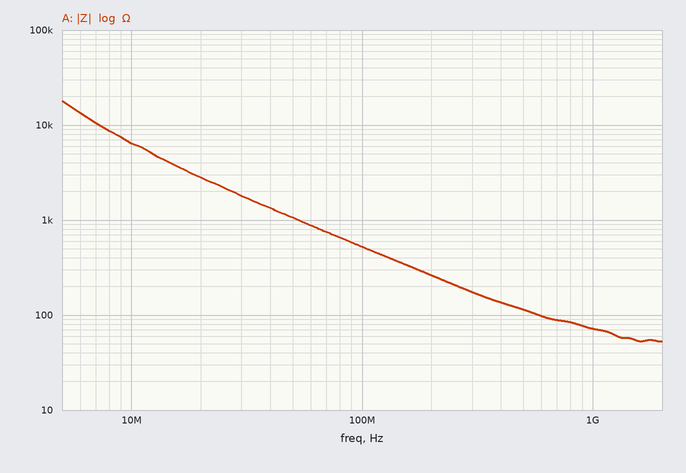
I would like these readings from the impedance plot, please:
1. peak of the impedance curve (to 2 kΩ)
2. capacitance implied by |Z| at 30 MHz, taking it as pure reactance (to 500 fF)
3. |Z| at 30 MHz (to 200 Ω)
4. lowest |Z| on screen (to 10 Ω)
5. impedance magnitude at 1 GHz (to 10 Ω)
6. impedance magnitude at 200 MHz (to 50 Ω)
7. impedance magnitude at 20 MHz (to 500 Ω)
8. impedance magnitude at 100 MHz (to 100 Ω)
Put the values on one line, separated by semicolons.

18 kΩ; 3.0 pF; 1.8 kΩ; 50 Ω; 70 Ω; 250 Ω; 3.0 kΩ; 500 Ω
